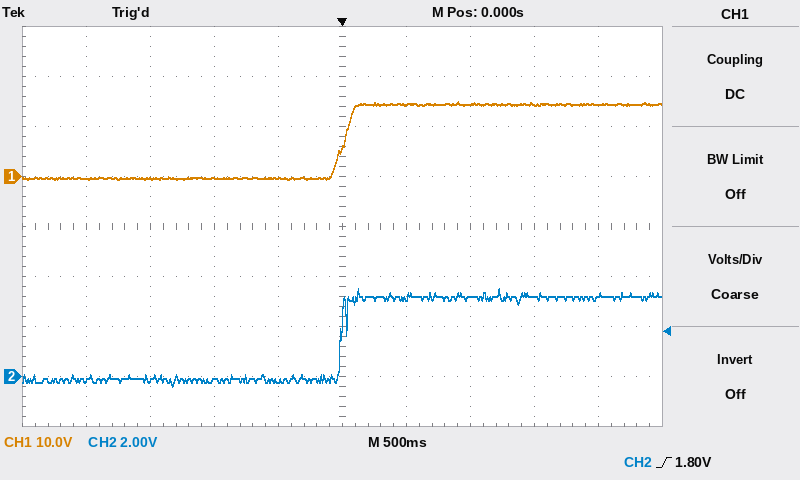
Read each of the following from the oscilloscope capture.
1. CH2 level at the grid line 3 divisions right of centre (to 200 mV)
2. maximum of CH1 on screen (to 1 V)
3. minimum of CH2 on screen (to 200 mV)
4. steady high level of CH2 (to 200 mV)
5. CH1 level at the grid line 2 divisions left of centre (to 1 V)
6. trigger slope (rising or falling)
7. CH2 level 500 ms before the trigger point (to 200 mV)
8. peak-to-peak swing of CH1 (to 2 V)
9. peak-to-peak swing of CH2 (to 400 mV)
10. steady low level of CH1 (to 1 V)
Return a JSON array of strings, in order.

["3.2 V", "15 V", "-400 mV", "3.2 V", "0 V", "rising", "-200 mV", "16 V", "4.0 V", "0 V"]
